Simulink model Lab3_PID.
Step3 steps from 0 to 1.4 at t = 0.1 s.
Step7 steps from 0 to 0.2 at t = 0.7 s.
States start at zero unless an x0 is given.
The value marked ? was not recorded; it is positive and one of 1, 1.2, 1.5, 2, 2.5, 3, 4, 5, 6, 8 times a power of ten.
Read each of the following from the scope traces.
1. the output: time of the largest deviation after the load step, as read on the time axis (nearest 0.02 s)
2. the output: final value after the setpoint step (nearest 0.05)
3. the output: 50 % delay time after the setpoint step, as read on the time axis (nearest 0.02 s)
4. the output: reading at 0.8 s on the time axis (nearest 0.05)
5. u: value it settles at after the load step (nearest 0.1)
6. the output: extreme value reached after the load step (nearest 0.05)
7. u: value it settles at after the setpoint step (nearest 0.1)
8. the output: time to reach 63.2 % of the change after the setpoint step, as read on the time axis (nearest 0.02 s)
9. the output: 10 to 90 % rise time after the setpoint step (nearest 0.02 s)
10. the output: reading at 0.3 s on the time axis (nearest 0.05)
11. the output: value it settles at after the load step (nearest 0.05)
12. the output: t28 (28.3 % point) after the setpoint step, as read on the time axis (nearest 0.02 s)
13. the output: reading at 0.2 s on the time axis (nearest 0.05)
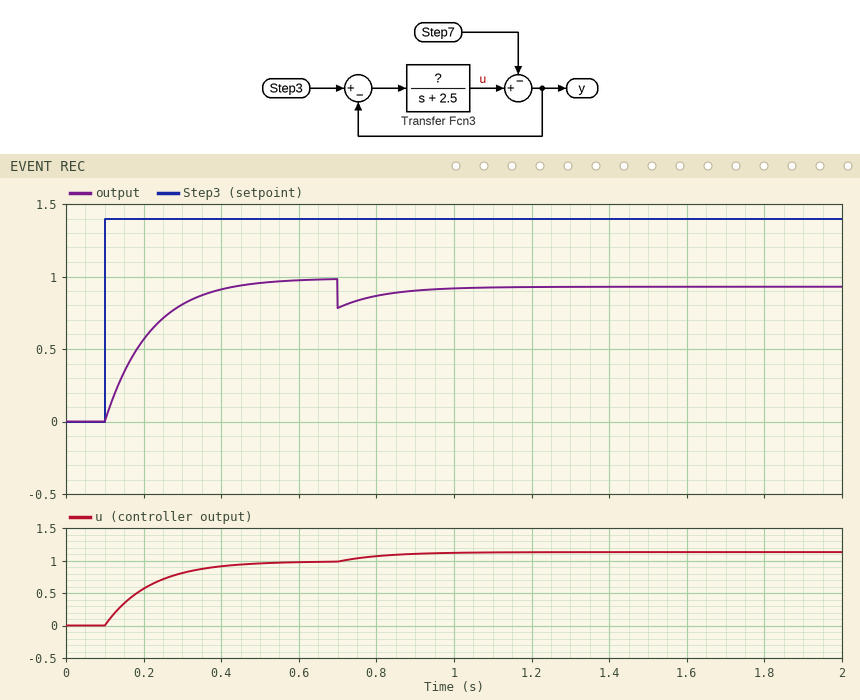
0.70 s
1.00
0.18 s
0.85
1.1
0.80
1.0
0.22 s
0.26 s
0.80
0.95
0.14 s
0.55
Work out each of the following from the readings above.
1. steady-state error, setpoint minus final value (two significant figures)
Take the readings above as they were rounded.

0.40
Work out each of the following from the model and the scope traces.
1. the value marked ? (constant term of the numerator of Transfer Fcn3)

6
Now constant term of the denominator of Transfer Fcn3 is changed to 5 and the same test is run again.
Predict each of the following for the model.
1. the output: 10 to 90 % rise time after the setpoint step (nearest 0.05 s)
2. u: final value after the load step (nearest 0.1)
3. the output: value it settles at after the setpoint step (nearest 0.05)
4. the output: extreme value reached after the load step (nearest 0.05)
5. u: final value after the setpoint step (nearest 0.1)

0.20 s
0.9
0.75
0.55
0.8
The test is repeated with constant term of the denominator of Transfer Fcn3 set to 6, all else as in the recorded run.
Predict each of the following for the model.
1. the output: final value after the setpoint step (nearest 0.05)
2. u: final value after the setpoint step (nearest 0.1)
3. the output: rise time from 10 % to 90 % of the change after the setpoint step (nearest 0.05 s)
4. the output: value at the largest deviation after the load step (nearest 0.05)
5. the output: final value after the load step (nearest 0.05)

0.70
0.7
0.20 s
0.50
0.60
